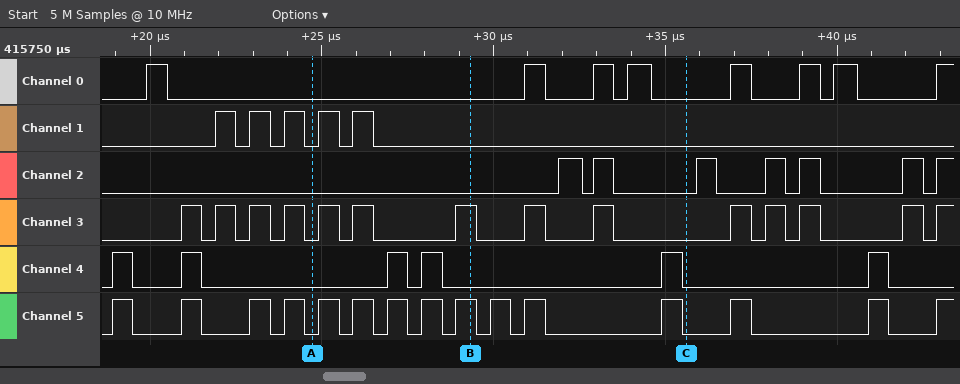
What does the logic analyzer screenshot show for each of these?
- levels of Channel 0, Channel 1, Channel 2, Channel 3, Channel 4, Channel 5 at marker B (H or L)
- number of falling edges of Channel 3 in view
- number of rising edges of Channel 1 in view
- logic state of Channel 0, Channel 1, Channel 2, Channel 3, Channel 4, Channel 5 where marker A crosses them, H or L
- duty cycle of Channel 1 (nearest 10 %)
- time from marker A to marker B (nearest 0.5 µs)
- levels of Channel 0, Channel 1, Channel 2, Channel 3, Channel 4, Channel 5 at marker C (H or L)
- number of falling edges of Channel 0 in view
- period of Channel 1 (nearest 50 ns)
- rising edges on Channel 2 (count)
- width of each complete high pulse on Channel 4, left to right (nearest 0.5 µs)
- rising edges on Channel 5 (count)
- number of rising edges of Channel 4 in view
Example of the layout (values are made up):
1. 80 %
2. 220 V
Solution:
1. Channel 0=L, Channel 1=L, Channel 2=L, Channel 3=H, Channel 4=L, Channel 5=H
2. 13
3. 5
4. Channel 0=L, Channel 1=L, Channel 2=L, Channel 3=L, Channel 4=L, Channel 5=L
5. 60 %
6. 4.5 µs
7. Channel 0=L, Channel 1=L, Channel 2=L, Channel 3=L, Channel 4=L, Channel 5=L
8. 7
9. 1000 ns
10. 7
11. 0.5 µs, 0.5 µs, 0.5 µs, 0.5 µs, 0.5 µs, 0.5 µs
12. 15
13. 6
